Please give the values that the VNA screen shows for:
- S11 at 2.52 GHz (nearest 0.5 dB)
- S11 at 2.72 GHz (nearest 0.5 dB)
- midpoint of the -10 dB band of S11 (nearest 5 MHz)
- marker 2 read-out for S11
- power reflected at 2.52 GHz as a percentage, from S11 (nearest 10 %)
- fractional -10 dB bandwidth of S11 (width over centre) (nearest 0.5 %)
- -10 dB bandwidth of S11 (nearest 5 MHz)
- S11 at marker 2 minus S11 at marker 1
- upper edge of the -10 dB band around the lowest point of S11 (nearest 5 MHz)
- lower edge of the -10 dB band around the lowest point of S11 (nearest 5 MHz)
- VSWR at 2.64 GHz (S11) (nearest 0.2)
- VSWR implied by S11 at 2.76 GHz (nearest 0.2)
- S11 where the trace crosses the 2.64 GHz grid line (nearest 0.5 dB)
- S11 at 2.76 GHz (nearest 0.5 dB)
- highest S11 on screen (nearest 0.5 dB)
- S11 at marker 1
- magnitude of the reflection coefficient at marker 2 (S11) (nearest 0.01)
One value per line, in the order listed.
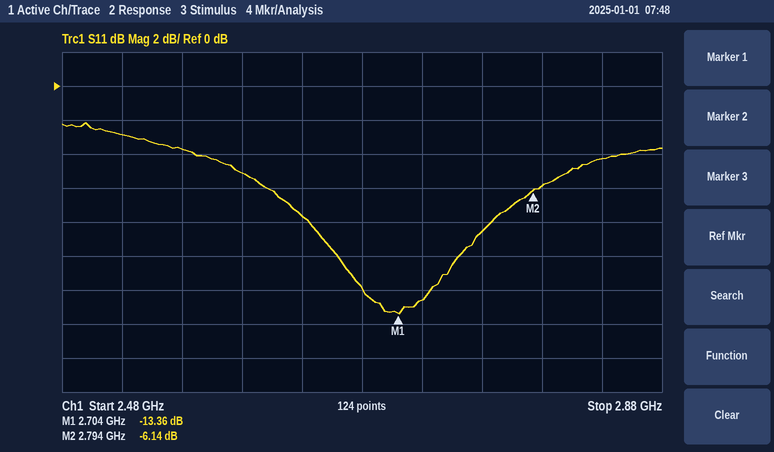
-3.0 dB
-12.5 dB
2.705 GHz
-6.14 dB
50 %
3.0 %
80 MHz
7.22 dB
2.745 GHz
2.665 GHz
2.4
2.2
-7.5 dB
-8.5 dB
-2.0 dB
-13.36 dB
0.49
